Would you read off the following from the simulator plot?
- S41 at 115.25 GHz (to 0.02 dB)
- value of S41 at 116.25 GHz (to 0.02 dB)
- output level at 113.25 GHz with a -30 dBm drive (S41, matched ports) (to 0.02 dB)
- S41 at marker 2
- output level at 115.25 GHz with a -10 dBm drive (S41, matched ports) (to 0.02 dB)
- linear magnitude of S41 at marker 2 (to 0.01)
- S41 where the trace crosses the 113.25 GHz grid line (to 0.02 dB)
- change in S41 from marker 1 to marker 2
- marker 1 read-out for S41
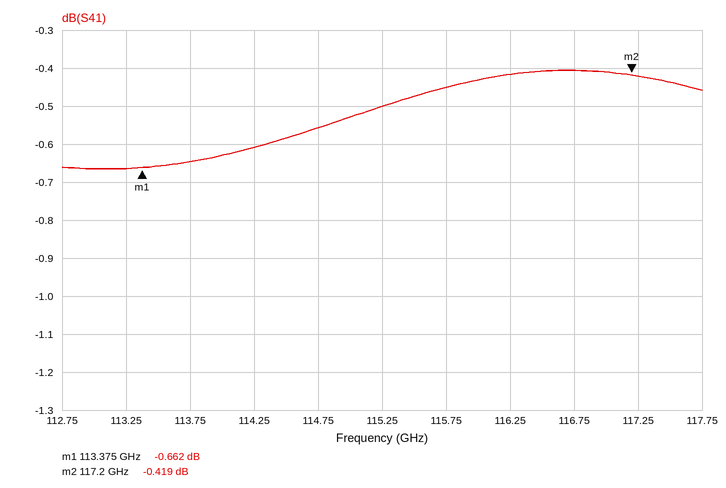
-0.50 dB
-0.42 dB
-30.66 dBm
-0.419 dB
-10.50 dBm
0.95
-0.66 dB
0.243 dB
-0.662 dB
